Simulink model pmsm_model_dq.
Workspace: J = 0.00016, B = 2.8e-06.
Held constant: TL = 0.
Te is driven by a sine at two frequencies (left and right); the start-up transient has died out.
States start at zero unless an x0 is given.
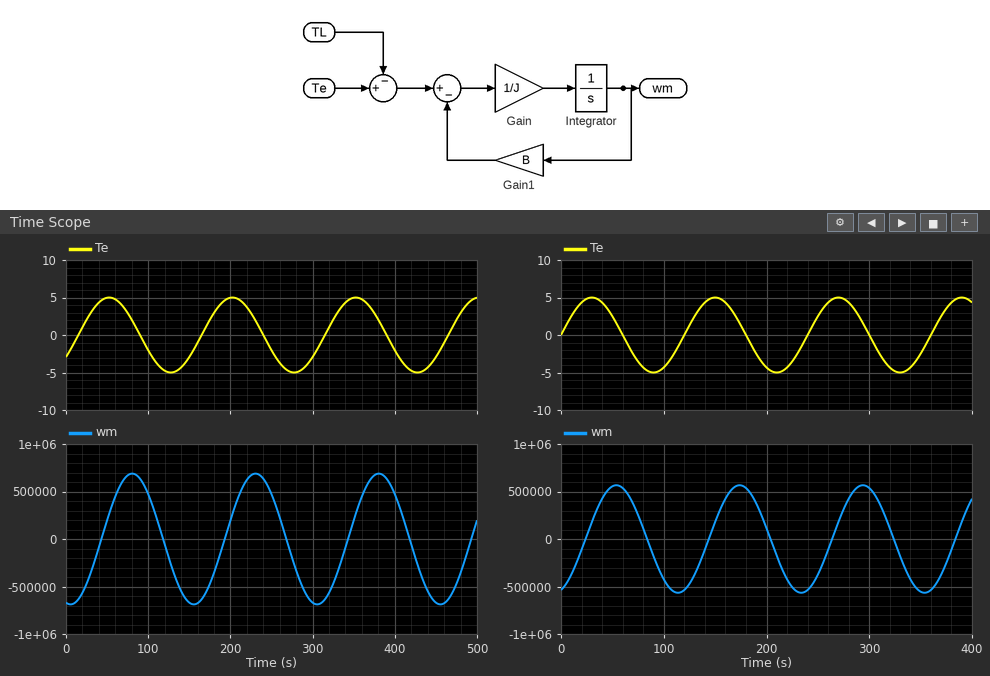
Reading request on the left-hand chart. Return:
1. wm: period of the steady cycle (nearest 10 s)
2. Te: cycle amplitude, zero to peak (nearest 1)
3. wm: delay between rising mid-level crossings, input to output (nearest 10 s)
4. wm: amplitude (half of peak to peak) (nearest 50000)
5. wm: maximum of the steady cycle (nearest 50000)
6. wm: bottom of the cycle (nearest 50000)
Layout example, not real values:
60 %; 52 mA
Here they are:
150 s; 5; 30 s; 700000; 700000; -700000
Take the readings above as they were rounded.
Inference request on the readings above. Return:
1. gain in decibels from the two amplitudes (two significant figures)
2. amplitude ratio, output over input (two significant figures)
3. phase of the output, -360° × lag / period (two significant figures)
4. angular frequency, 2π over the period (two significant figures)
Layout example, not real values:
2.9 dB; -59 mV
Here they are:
100 dB; 140000; -72°; 0.042 rad/s
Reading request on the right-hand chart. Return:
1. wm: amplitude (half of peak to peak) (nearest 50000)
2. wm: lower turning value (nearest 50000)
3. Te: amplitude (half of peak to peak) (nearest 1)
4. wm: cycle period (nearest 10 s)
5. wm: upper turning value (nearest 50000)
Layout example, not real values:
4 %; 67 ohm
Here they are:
550000; -550000; 5; 120 s; 550000
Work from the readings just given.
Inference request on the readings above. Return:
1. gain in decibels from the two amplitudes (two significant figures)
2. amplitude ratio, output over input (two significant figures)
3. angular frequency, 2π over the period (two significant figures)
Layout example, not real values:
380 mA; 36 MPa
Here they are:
100 dB; 110000; 0.052 rad/s
